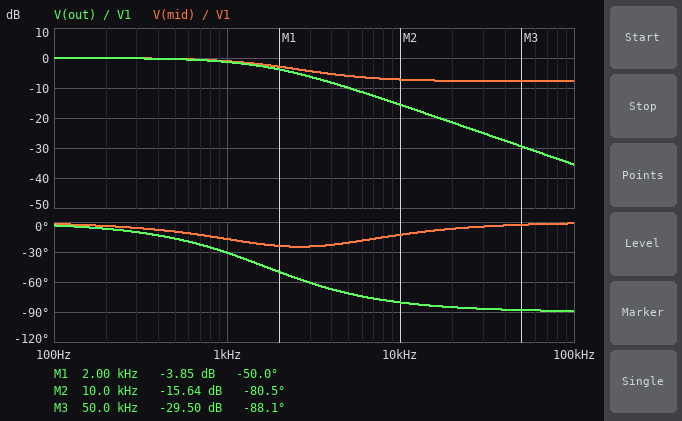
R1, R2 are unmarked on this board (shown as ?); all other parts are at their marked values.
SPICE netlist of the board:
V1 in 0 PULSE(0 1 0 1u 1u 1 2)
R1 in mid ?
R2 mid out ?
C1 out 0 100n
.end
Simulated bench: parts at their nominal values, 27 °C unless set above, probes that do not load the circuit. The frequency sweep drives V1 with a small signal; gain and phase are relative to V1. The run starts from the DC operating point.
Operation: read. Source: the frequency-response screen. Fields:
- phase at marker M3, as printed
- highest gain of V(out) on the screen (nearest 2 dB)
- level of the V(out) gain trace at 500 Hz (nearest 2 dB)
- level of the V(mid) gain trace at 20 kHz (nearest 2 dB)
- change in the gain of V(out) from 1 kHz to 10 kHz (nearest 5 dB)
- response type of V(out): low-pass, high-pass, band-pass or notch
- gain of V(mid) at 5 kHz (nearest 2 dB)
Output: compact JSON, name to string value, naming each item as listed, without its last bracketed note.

{"phase at marker M3, as printed": "-88.1 deg", "highest gain of V(out) on the screen": "0 dB", "level of the V(out) gain trace at 500 Hz": "0 dB", "level of the V(mid) gain trace at 20 kHz": "-8 dB", "change in the gain of V(out) from 1 kHz to 10 kHz": "-15 dB", "response type of V(out): low-pass, high-pass, band-pass or notch": "low-pass", "gain of V(mid) at 5 kHz": "-6 dB"}
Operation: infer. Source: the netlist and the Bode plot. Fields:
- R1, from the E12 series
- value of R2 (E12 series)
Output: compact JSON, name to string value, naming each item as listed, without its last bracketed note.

{"R1, from the E12 series": "560 Ω", "value of R2": "390 Ω"}
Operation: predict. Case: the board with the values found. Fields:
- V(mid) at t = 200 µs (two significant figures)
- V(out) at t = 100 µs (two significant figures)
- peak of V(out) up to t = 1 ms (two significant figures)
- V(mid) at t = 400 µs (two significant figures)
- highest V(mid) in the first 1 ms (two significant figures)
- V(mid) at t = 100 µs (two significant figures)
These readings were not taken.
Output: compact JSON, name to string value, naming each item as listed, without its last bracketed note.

{"V(mid) at t = 200 µs": "930 mV", "V(out) at t = 100 µs": "650 mV", "peak of V(out) up to t = 1 ms": "1.0 V", "V(mid) at t = 400 µs": "990 mV", "highest V(mid) in the first 1 ms": "1.0 V", "V(mid) at t = 100 µs": "790 mV"}
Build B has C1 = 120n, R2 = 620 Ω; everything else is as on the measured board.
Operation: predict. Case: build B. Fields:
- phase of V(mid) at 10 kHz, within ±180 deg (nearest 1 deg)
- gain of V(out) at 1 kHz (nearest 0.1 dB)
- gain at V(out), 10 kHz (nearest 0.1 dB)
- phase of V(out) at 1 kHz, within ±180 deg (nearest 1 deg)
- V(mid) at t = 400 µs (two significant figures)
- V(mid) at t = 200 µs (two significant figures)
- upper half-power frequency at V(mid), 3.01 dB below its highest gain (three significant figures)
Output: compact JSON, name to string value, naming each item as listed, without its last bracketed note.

{"phase of V(mid) at 10 kHz, within ±180 deg": "-6 deg", "gain of V(out) at 1 kHz": "-2.5 dB", "gain at V(out), 10 kHz": "-19.0 dB", "phase of V(out) at 1 kHz, within ±180 deg": "-42 deg", "V(mid) at t = 400 µs": "970 mV", "V(mid) at t = 200 µs": "880 mV", "upper half-power frequency at V(mid), 3.01 dB below its highest gain": "1.68 kHz"}
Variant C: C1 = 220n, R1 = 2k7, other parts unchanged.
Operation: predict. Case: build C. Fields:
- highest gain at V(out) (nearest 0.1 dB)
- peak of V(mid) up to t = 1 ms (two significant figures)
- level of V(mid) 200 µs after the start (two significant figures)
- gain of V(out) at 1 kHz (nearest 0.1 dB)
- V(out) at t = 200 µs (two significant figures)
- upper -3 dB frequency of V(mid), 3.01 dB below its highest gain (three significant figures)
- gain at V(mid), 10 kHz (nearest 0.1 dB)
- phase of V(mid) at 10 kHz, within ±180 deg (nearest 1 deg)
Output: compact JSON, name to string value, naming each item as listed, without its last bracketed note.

{"highest gain at V(out)": "0 dB", "peak of V(mid) up to t = 1 ms": "800 mV", "level of V(mid) 200 µs after the start": "350 mV", "gain of V(out) at 1 kHz": "-12.8 dB", "V(out) at t = 200 µs": "250 mV", "upper -3 dB frequency of V(mid), 3.01 dB below its highest gain": "238 Hz", "gain at V(mid), 10 kHz": "-17.8 dB", "phase of V(mid) at 10 kHz, within ±180 deg": "-9 deg"}
